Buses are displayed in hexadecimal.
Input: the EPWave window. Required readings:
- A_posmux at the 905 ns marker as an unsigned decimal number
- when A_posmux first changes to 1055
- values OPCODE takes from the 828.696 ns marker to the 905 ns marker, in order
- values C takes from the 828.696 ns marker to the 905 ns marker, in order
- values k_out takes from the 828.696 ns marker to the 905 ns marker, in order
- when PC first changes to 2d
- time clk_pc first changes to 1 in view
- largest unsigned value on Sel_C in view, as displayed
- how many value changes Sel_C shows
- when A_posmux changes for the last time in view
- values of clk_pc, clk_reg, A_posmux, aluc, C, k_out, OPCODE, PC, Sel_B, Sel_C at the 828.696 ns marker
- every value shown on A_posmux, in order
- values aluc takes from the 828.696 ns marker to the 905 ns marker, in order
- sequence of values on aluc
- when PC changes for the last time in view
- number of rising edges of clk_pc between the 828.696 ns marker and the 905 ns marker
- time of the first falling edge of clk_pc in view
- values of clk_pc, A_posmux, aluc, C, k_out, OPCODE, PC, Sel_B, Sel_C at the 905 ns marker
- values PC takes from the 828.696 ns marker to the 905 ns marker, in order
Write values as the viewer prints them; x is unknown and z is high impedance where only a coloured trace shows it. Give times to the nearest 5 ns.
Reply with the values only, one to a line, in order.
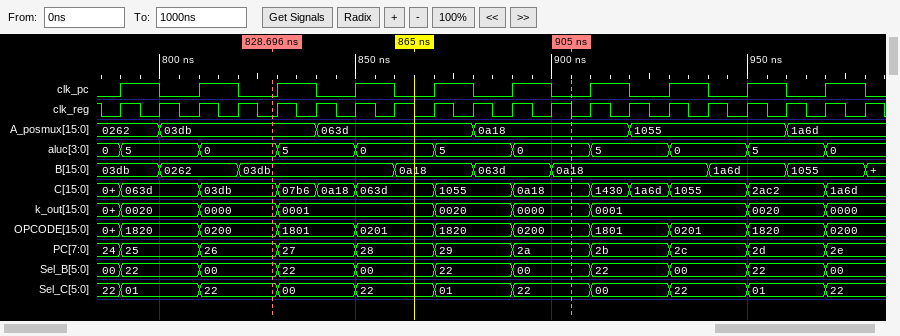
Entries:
2584
920 ns
0200, 1801, 0201, 1820, 0200
03db, 07b6, 0a18, 063d, 1055, 0a18
0000, 0001, 0020, 0000
950 ns
790 ns
22
10
960 ns
clk_pc=0, clk_reg=0, A_posmux=03db, aluc=0, C=03db, k_out=0000, OPCODE=0200, PC=26, Sel_B=00, Sel_C=22
0262, 03db, 063d, 0a18, 1055, 1a6d
0, 5, 0, 5, 0
0, 5, 0, 5, 0, 5, 0, 5, 0, 5, 0
970 ns
4
800 ns
clk_pc=0, A_posmux=0a18, aluc=0, C=0a18, k_out=0000, OPCODE=0200, PC=2a, Sel_B=00, Sel_C=22
26, 27, 28, 29, 2a
